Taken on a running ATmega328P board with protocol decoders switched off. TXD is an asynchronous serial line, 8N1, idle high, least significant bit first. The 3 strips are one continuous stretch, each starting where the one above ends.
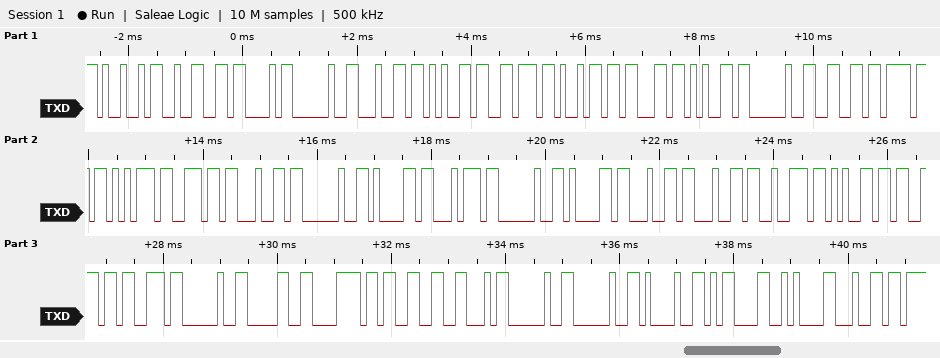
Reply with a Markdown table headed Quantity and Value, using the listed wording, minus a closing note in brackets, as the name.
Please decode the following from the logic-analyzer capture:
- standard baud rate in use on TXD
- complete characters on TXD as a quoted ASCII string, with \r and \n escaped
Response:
| Quantity | Value |
|---|---|
| standard baud rate in use on TXD | 9600 baud |
| complete characters on TXD as a quoted ASCII string, with \r and \n escaped | "I2C device found at address 0x3F  !\r\nd" |
